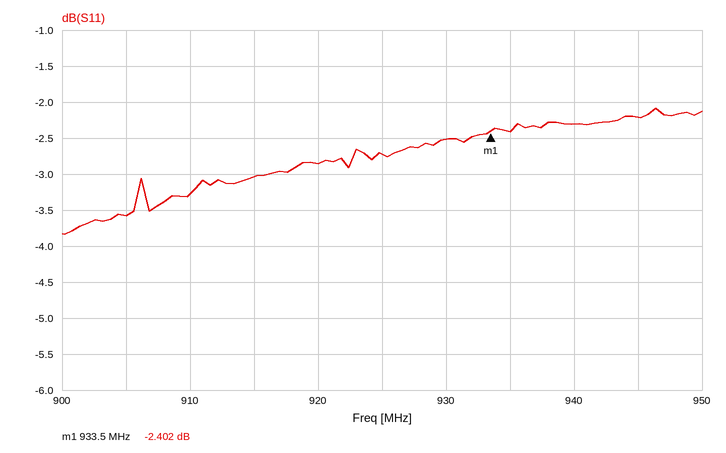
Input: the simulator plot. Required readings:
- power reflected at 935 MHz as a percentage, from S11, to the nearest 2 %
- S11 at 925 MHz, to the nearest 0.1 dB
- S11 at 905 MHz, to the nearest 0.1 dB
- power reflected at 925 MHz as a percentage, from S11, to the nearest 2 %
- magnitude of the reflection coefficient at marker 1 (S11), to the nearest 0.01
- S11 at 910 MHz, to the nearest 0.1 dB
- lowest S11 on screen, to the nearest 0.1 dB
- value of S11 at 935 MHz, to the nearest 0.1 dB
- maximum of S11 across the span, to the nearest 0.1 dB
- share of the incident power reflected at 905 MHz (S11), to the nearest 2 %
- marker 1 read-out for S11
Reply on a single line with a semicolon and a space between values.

58 %; -2.7 dB; -3.6 dB; 54 %; 0.76; -3.3 dB; -3.8 dB; -2.4 dB; -2.1 dB; 44 %; -2.402 dB
